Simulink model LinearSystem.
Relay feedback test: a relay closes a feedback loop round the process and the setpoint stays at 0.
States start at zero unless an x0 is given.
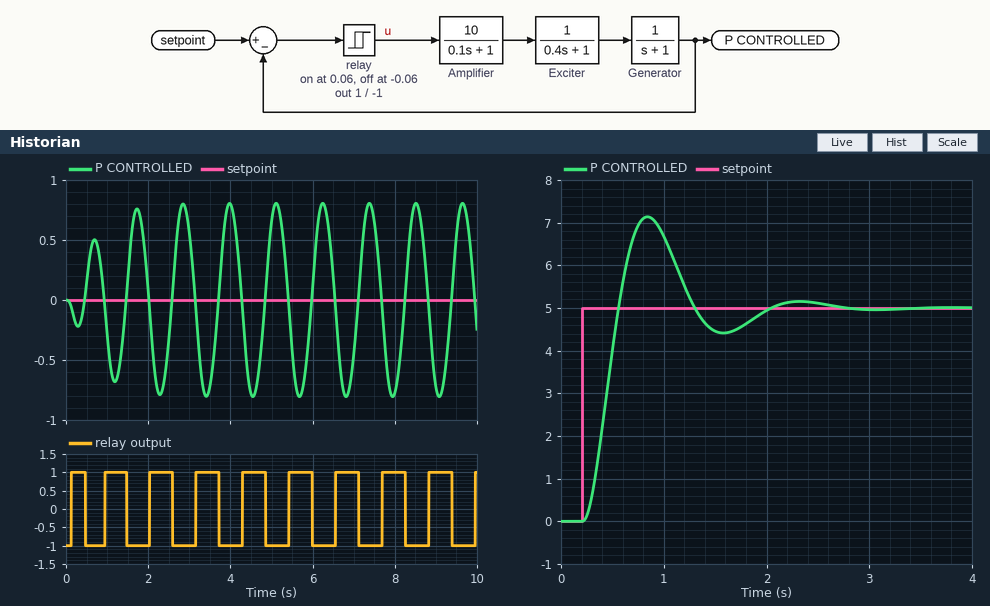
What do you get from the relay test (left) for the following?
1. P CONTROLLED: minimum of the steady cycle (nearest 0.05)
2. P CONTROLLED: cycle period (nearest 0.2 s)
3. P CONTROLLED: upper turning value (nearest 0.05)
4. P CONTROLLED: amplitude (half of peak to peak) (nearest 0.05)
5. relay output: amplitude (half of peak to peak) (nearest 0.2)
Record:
-0.80
1.2 s
0.80
0.80
1.0
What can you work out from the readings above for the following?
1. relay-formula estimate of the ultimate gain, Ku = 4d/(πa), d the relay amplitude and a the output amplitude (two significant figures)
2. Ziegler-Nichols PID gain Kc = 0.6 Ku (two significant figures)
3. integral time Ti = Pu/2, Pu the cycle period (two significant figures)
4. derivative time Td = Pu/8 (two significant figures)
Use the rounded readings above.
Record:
1.6
0.96
0.60 s
0.15 s
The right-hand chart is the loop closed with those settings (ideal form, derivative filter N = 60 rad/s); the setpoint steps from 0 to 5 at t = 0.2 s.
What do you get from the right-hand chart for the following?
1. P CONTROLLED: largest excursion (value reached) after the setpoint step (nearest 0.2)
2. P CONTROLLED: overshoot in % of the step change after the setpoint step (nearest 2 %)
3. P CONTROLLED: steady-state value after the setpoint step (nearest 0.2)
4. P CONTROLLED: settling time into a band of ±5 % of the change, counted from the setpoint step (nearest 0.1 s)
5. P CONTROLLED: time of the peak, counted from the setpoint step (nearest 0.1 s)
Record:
7.2
42 %
5.0
1.7 s
0.6 s
